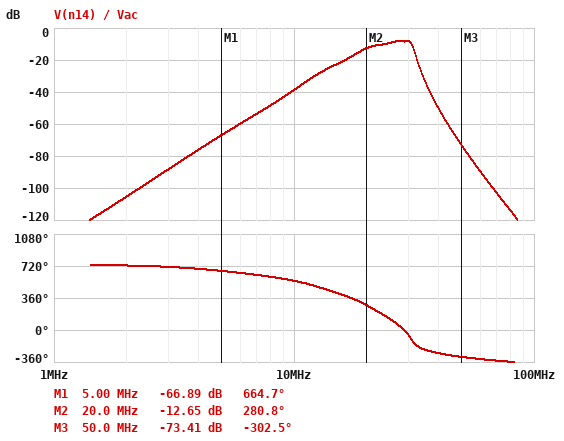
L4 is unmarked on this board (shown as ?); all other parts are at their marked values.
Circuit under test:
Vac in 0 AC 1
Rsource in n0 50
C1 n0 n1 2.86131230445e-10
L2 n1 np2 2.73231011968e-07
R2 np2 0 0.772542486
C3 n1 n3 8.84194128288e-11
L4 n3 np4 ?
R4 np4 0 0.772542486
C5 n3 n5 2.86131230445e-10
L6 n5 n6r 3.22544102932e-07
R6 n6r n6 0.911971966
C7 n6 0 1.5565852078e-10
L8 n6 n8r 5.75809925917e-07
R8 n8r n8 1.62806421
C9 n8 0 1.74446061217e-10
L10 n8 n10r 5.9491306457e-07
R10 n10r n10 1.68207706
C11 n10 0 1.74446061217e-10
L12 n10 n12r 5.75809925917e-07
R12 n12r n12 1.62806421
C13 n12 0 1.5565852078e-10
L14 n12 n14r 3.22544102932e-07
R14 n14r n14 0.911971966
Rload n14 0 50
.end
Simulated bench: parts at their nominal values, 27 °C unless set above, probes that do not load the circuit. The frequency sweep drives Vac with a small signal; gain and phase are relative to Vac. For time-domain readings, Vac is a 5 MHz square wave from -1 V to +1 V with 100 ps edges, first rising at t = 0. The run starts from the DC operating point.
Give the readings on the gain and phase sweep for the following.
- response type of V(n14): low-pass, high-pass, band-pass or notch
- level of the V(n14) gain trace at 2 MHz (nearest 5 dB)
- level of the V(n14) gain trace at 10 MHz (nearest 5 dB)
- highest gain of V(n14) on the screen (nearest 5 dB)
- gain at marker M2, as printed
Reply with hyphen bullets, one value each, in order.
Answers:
- band-pass
- -105 dB
- -40 dB
- -10 dB
- -12.65 dB
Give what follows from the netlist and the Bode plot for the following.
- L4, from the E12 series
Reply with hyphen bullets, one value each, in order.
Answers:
- 150 nH
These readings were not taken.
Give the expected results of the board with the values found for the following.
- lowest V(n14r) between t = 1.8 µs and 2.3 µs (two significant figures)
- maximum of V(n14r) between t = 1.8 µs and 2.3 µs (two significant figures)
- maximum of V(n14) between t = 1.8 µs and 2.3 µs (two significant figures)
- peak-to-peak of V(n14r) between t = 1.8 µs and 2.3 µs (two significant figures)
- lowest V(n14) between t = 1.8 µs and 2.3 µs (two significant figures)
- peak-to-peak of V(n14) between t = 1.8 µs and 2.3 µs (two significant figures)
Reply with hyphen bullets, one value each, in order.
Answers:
- -120 mV
- 120 mV
- 120 mV
- 240 mV
- -120 mV
- 240 mV
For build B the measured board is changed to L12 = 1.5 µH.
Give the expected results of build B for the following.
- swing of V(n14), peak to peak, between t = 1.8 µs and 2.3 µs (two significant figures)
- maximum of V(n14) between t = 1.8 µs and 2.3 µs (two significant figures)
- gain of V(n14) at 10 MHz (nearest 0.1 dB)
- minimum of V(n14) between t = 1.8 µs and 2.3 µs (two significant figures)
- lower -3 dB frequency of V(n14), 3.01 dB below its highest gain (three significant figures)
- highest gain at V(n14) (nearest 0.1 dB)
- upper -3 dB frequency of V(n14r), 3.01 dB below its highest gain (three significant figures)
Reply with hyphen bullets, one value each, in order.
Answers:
- 120 mV
- 61 mV
- -40.8 dB
- -61 mV
- 21.8 MHz
- -9.5 dB
- 23.8 MHz
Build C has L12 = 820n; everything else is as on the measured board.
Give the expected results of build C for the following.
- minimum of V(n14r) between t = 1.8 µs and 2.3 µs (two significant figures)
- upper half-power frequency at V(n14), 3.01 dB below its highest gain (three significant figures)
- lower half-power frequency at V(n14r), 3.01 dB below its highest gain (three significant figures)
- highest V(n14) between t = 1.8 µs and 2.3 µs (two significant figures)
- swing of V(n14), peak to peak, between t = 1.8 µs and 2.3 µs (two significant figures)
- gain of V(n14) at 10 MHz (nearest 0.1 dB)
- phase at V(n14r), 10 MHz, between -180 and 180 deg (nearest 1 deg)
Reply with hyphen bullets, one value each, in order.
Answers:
- -130 mV
- 26.5 MHz
- 21.8 MHz
- 130 mV
- 250 mV
- -39.3 dB
- -168 deg
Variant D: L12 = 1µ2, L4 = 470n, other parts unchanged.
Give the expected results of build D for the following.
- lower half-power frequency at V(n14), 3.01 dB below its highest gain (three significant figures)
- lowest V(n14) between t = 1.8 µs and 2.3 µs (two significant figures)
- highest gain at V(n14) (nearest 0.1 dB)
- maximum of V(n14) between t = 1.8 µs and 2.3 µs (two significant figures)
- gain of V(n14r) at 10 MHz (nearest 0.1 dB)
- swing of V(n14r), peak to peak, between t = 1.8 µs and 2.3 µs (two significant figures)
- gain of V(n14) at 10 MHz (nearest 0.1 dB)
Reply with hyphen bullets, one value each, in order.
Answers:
- 17.3 MHz
- -130 mV
- -7.4 dB
- 130 mV
- -25.3 dB
- 260 mV
- -25.4 dB
